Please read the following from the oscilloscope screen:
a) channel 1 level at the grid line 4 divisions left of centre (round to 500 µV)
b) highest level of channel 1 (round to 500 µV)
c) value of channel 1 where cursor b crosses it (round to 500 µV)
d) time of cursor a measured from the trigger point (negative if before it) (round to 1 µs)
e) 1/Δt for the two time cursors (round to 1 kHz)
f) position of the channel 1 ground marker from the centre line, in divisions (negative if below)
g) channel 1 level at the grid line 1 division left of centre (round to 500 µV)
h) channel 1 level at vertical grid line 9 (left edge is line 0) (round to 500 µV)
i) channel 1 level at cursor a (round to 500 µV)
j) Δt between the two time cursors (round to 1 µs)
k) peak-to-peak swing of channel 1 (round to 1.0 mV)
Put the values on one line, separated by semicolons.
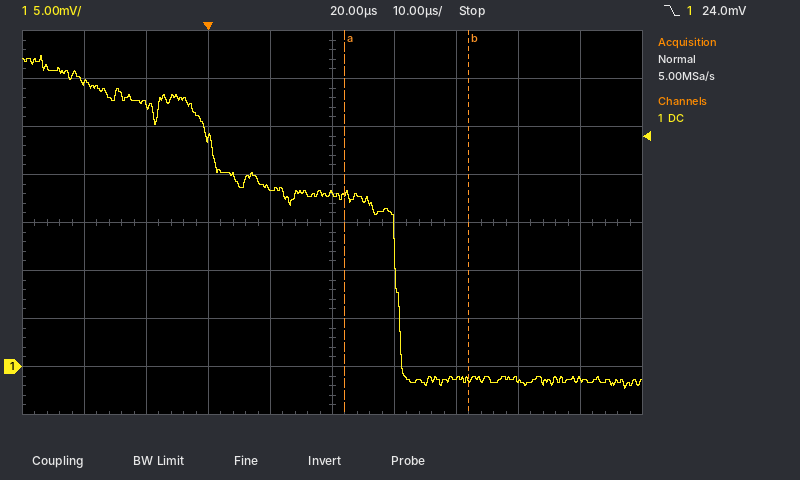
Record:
29.5 mV; 32.5 mV; -1.5 mV; +22 µs; 50 kHz; -3.0 div; 18.5 mV; -1.5 mV; 18.0 mV; 20 µs; 35.0 mV
